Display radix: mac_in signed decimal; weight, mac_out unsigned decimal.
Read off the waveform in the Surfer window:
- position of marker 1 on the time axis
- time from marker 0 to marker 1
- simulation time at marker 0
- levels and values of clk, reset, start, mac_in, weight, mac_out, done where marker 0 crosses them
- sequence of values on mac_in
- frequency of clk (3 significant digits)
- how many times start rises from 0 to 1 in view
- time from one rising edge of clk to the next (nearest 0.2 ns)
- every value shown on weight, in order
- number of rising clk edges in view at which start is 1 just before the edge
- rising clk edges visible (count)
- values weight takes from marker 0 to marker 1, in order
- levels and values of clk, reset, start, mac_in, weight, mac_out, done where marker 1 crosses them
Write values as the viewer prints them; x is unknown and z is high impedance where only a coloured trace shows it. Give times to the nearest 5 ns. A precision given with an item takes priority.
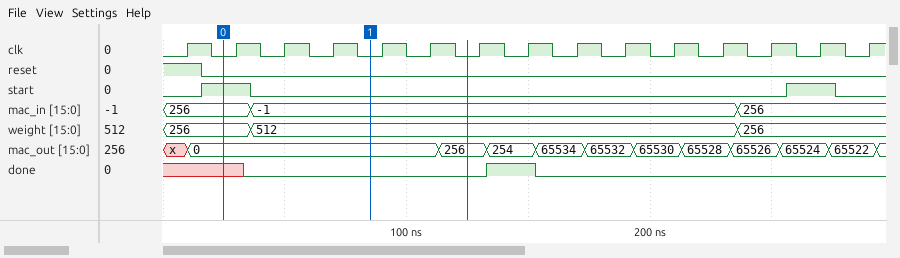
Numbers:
85 ns
60 ns
25 ns
clk=0, reset=0, start=1, mac_in=256, weight=256, mac_out=0, done=x
256, -1, 256
50.0 MHz
2
20 ns
256, 512, 256
2
15
256, 512
clk=0, reset=0, start=0, mac_in=-1, weight=512, mac_out=0, done=0
